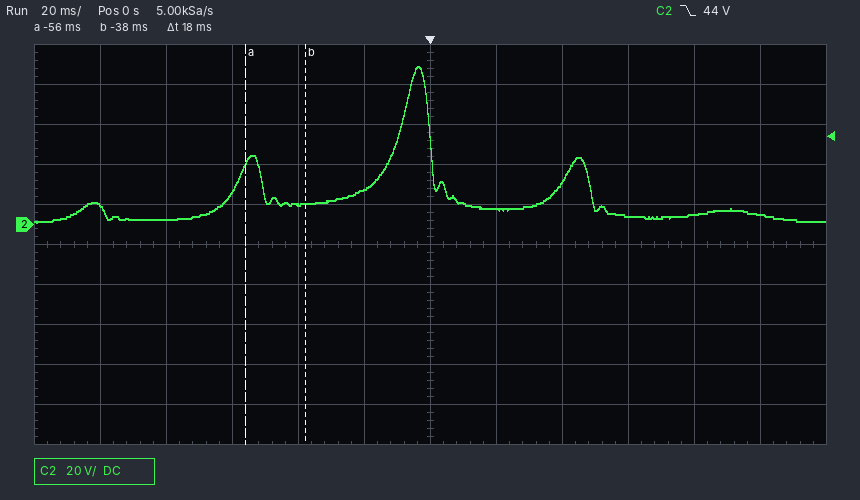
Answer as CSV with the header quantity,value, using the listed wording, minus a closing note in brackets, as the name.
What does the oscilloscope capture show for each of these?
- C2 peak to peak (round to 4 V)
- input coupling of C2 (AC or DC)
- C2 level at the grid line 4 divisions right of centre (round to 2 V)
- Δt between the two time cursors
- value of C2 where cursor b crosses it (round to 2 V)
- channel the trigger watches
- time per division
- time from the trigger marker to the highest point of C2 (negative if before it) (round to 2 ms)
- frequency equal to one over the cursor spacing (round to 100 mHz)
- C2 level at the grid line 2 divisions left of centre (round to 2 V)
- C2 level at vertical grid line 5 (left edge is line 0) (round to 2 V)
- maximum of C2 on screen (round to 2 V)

quantity,value
C2 peak to peak,80 V
input coupling of C2,DC
C2 level at the grid line 4 divisions right of centre,4 V
Δt between the two time cursors,18 ms
value of C2 where cursor b crosses it,10 V
channel the trigger watches,C2
time per division,20 ms
time from the trigger marker to the highest point of C2 (negative if before it),-4 ms
frequency equal to one over the cursor spacing,55.6 Hz
C2 level at the grid line 2 divisions left of centre,10 V
C2 level at vertical grid line 5 (left edge is line 0),18 V
maximum of C2 on screen,80 V
